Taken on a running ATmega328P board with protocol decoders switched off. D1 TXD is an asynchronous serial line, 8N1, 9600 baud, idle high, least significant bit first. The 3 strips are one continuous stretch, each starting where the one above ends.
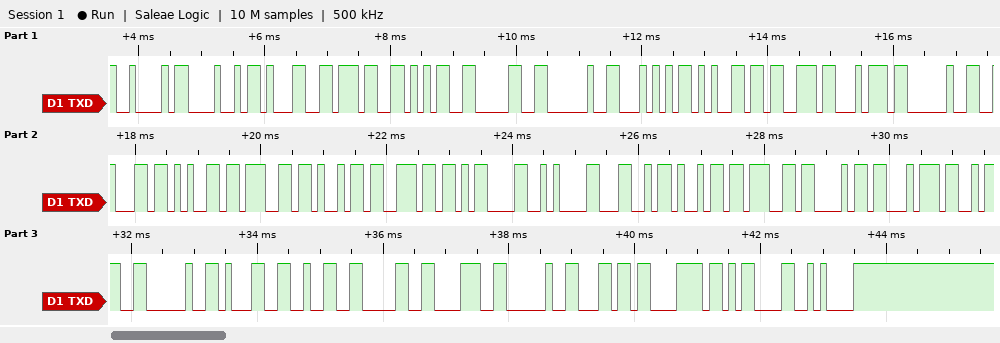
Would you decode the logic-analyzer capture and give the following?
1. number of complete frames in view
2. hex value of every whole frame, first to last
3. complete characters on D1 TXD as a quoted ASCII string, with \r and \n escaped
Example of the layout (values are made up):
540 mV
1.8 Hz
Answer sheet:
35
42 48 31 37 35 30 20 54 65 73 74 20 62 65 67 69 6E 0D 0A 4C 69 67 68 74 3A 20 31 32 30 38 20 6C 78 0D 0A
"BH1750 Test begin\r\nLight: 1208 lx\r\n"
